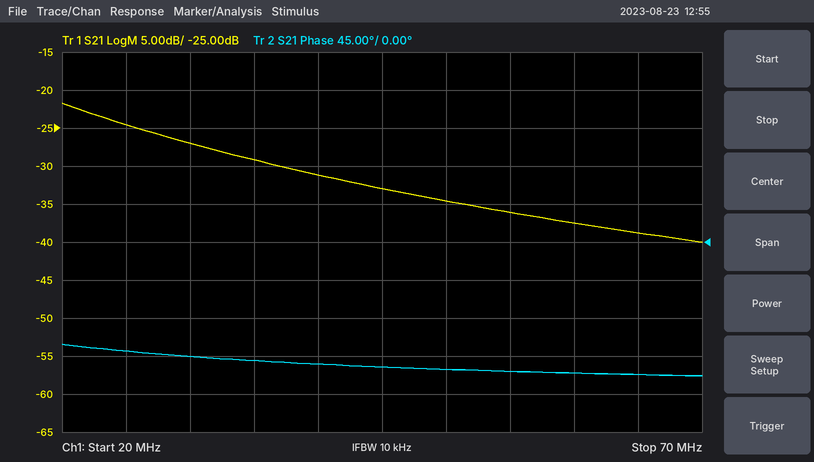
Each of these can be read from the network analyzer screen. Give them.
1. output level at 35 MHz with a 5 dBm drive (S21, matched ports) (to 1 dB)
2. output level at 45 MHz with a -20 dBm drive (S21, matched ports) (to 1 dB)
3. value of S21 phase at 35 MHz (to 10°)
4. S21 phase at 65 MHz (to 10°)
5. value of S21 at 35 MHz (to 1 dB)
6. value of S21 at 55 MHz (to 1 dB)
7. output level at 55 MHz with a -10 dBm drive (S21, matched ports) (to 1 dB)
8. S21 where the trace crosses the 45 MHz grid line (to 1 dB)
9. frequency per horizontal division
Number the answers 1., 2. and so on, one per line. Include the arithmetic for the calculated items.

1. 5 dBm + (-29 dB) = -24 dBm
2. -20 dBm + (-33 dB) = -53 dBm
3. -140°
4. -160°
5. -29 dB
6. -36 dB
7. -10 dBm + (-36 dB) = -46 dBm
8. -33 dB
9. 5 MHz
